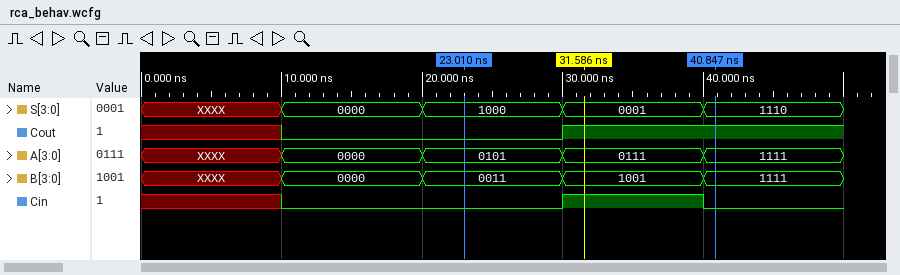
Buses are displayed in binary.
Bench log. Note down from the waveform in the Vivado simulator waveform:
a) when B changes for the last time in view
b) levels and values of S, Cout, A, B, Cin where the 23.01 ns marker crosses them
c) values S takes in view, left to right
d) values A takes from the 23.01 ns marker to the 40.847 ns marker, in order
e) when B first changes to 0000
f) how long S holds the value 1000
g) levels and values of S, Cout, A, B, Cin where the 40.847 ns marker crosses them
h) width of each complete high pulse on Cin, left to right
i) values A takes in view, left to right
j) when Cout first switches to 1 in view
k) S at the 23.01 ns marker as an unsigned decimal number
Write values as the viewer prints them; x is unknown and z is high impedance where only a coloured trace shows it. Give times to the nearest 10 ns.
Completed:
40 ns
S=1000, Cout=0, A=0101, B=0011, Cin=0
XXXX, 0000, 1000, 0001, 1110
0101, 0111, 1111
10 ns
10 ns
S=1110, Cout=1, A=1111, B=1111, Cin=0
10 ns
XXXX, 0000, 0101, 0111, 1111
30 ns
8
